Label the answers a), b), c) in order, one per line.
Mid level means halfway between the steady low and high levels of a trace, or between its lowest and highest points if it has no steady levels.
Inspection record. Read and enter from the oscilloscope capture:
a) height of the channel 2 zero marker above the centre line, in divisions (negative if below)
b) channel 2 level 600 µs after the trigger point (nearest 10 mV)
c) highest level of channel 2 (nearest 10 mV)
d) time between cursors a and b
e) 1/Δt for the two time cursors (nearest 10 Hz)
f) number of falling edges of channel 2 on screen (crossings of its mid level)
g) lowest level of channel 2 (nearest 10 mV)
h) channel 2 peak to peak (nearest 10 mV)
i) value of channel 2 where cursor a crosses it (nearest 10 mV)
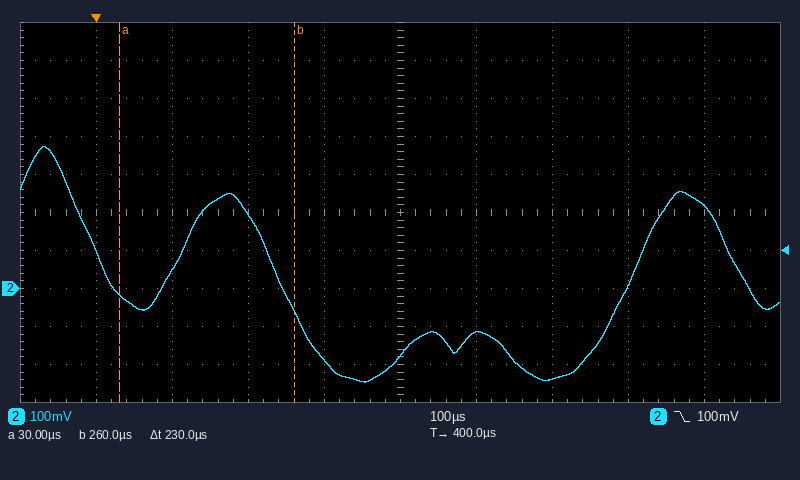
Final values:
a) -2.0 div
b) -240 mV
c) 370 mV
d) 230 µs
e) 4.35 kHz
f) 3
g) -250 mV
h) 620 mV
i) -20 mV
